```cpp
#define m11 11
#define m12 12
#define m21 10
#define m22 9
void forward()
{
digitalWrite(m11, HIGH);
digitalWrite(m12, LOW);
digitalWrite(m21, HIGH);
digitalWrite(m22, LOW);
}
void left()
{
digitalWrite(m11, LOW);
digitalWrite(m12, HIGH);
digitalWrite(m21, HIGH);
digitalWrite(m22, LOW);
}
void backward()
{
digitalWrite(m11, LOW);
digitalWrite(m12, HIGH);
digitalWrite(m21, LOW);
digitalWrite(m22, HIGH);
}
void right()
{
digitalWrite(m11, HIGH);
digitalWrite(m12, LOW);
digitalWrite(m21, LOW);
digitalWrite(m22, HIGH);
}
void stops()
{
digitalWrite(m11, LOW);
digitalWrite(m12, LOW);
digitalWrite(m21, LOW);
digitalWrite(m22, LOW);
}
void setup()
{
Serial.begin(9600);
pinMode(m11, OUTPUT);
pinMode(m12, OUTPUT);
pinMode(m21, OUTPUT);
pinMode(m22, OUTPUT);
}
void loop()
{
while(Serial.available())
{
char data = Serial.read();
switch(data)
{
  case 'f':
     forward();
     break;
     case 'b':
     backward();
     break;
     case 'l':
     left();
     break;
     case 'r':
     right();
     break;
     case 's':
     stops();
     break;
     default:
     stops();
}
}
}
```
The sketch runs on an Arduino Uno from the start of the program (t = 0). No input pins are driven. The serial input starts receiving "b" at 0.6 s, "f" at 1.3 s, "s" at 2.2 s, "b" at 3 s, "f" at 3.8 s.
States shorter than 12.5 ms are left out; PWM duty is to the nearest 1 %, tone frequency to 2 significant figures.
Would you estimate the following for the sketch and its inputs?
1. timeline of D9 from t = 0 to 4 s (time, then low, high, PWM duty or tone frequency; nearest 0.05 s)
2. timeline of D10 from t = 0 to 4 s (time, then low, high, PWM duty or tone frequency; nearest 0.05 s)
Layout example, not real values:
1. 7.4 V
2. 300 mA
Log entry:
1. 0 s low; 0.6 s high; 1.3 s low; 3 s high; 3.8 s low
2. 0 s low; 1.3 s high; 2.2 s low; 3.8 s high
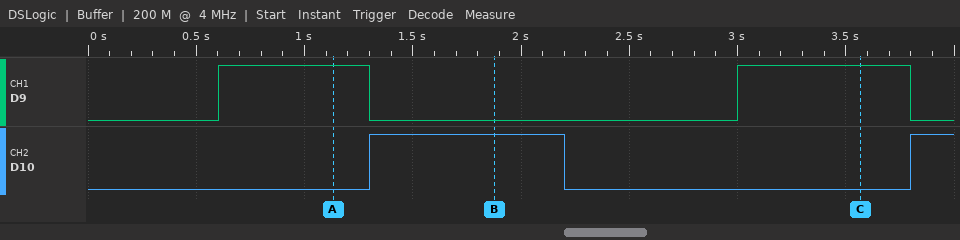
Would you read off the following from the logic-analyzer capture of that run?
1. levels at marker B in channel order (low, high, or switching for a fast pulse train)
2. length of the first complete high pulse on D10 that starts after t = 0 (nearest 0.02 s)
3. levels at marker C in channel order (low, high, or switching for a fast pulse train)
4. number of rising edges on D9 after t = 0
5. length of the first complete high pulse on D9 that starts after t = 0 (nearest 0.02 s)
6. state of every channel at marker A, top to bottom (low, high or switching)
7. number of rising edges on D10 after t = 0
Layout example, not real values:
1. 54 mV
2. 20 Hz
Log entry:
1. D9 low, D10 high
2. 0.90 s
3. D9 high, D10 low
4. 2
5. 0.70 s
6. D9 high, D10 low
7. 2
